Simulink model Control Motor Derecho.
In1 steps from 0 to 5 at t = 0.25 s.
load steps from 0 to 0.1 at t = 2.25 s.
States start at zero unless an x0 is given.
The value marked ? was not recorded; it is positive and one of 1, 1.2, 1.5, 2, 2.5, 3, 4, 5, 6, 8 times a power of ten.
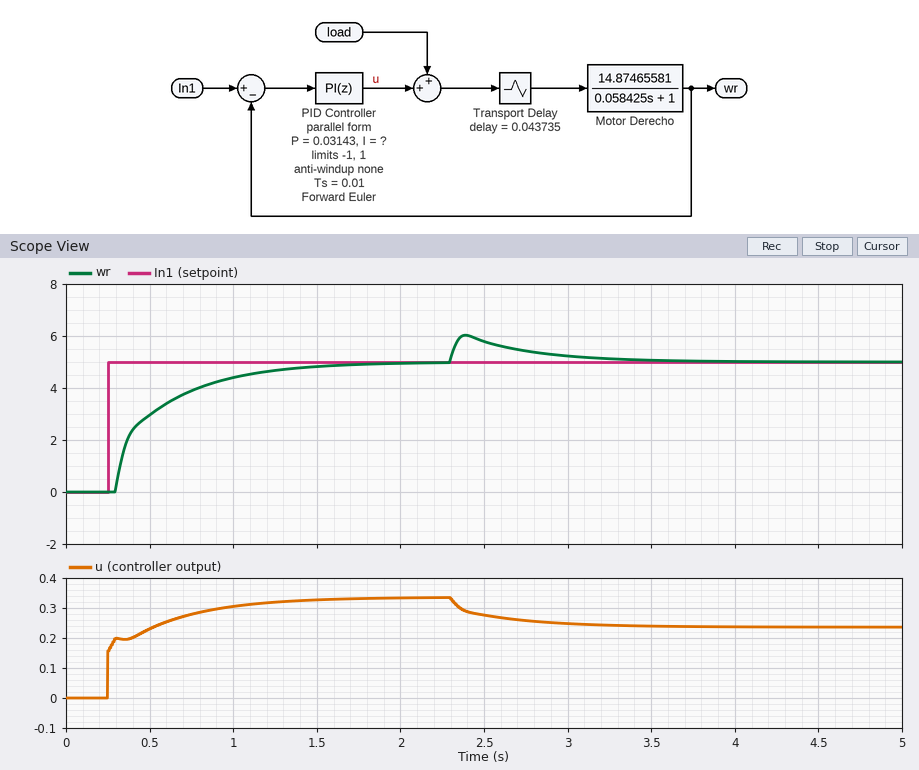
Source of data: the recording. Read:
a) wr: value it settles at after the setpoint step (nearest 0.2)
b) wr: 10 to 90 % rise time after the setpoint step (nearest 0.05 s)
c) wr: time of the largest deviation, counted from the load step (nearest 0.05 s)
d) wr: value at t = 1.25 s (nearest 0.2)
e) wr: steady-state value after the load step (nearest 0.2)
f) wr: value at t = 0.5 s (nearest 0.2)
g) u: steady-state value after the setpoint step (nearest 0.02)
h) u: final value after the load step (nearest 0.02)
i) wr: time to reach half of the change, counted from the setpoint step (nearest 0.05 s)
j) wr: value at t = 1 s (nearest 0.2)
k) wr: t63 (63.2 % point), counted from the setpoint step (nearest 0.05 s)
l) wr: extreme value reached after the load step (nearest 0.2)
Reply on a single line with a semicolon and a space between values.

5.0; 0.75 s; 0.15 s; 4.6; 5.0; 3.0; 0.34; 0.24; 0.15 s; 4.4; 0.30 s; 6.0
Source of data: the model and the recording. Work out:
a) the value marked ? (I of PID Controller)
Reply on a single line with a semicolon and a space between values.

0.2
